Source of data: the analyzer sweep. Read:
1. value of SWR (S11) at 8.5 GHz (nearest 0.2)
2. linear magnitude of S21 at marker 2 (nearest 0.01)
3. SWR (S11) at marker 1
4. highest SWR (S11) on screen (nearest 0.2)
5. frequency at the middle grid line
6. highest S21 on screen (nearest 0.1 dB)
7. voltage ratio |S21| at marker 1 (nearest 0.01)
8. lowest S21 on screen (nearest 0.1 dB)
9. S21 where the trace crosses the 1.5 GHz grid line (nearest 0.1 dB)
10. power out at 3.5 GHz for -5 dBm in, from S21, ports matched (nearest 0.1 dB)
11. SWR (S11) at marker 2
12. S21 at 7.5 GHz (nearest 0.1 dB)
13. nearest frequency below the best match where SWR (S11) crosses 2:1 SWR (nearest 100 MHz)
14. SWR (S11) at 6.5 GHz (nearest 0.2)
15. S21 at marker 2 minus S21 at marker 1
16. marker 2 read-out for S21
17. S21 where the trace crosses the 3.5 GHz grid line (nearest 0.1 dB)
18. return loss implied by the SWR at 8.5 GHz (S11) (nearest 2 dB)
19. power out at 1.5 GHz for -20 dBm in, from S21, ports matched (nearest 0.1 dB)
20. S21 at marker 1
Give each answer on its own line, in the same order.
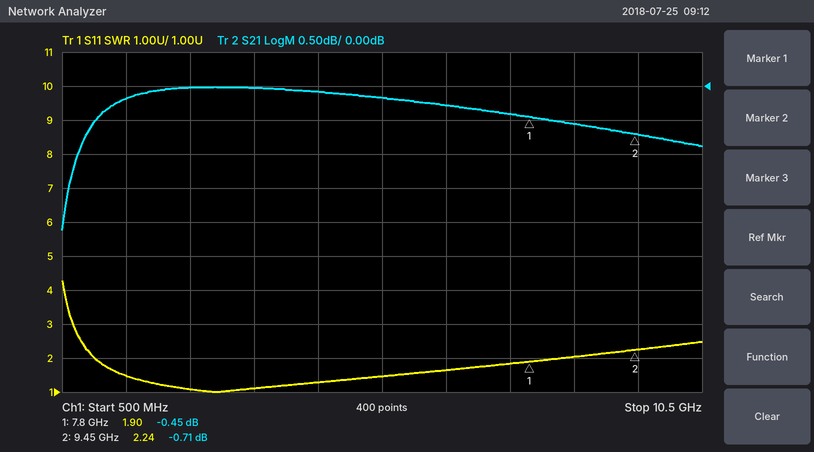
2.0
0.92
1.90
4.2
5.5 GHz
0.0 dB
0.95
-2.1 dB
-0.2 dB
-5.0 dBm
2.24
-0.4 dB
1.0 GHz
1.6
-0.26 dB
-0.71 dB
0.0 dB
10 dB
-20.2 dBm
-0.45 dB
